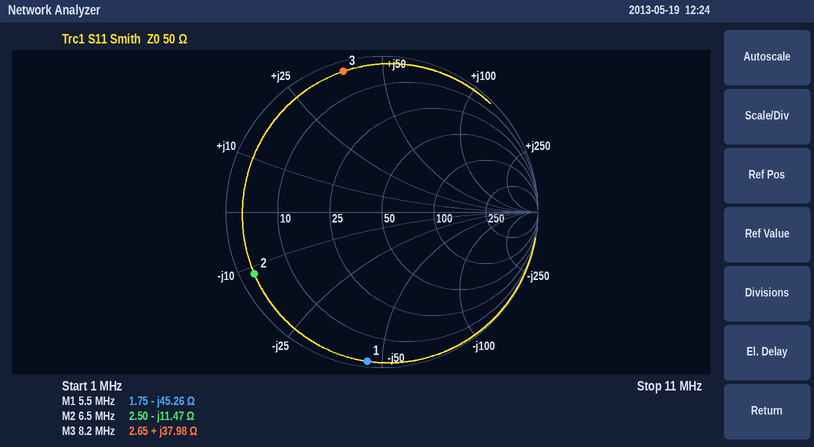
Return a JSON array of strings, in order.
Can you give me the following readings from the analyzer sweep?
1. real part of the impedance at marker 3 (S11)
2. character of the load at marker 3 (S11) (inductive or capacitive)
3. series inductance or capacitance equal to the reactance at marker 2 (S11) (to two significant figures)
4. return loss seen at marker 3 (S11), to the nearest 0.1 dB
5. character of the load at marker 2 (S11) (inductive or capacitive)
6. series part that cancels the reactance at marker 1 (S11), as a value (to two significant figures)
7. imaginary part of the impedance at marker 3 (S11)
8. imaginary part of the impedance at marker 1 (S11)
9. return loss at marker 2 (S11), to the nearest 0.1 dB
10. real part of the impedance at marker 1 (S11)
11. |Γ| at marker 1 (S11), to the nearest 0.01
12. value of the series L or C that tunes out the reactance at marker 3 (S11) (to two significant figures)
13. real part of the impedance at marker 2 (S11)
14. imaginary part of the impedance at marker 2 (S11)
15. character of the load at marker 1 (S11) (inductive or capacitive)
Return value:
["2.65 Ω", "inductive", "2.1 nF", "0.6 dB", "capacitive", "1.3 µH", "+37.98 Ω", "-45.26 Ω", "0.8 dB", "1.75 Ω", "0.96", "510 pF", "2.50 Ω", "-11.47 Ω", "capacitive"]
